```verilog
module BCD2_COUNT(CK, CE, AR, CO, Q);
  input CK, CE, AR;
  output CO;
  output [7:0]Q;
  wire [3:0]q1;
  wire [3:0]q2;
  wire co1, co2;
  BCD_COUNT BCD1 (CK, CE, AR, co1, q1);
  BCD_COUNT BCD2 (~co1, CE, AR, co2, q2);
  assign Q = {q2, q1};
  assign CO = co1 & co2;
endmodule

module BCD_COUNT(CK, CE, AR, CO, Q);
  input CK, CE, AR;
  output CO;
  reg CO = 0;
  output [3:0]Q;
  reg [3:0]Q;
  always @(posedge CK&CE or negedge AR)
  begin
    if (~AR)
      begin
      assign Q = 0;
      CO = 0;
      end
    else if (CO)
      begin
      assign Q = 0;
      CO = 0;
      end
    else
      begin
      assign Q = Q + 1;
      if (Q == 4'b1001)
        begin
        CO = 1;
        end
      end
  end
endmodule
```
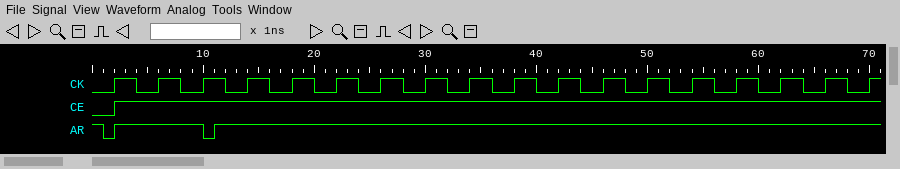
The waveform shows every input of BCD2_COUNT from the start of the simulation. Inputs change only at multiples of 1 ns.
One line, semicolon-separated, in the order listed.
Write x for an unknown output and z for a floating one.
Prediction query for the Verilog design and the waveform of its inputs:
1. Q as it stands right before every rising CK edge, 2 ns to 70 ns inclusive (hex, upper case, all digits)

00, 11, 12, 00, 01, 02, 03, 04, 05, 06, 07, 08, 09, 10, 11, 12, 13, 14
